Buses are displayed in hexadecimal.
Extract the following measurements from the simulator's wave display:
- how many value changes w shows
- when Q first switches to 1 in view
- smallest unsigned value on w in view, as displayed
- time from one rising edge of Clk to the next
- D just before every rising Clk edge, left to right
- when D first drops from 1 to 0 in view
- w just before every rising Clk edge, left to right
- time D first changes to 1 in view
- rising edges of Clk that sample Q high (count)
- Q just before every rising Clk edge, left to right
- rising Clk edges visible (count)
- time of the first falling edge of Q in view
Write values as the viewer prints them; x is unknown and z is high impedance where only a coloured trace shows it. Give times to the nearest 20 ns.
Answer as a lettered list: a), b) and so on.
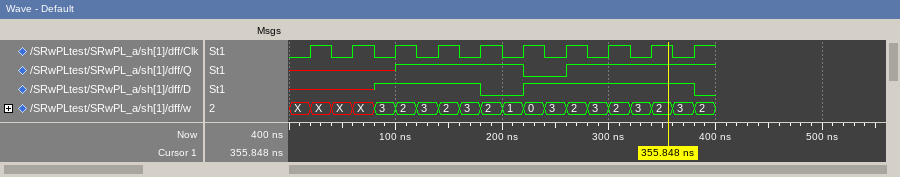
a) 19
b) 100 ns
c) 0
d) 40 ns
e) x x 1 1 1 0 1 1 1 1
f) 180 ns
g) X, X, 3, 3, 3, 1, 3, 3, 3, 3
h) 80 ns
i) 6
j) x x x 1 1 1 0 1 1 1
k) 10
l) 220 ns
